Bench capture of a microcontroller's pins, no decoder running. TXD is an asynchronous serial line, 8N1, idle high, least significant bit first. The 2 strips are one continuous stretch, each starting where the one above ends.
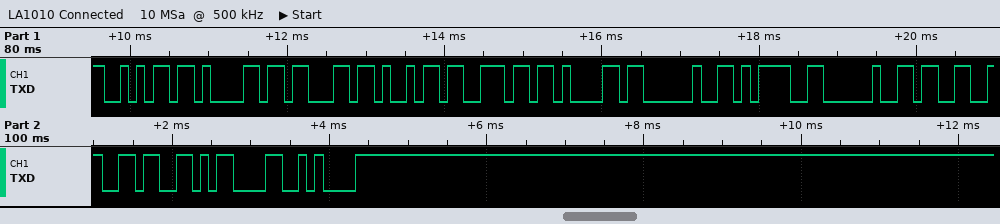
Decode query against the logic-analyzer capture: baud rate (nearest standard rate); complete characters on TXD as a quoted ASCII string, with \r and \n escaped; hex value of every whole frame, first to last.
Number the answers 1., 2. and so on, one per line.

1. 9600 baud
2. "jacina = 36\r\n"
3. 0x6A 0x61 0x63 0x69 0x6E 0x61 0x20 0x3D 0x20 0x33 0x36 0x0D 0x0A
